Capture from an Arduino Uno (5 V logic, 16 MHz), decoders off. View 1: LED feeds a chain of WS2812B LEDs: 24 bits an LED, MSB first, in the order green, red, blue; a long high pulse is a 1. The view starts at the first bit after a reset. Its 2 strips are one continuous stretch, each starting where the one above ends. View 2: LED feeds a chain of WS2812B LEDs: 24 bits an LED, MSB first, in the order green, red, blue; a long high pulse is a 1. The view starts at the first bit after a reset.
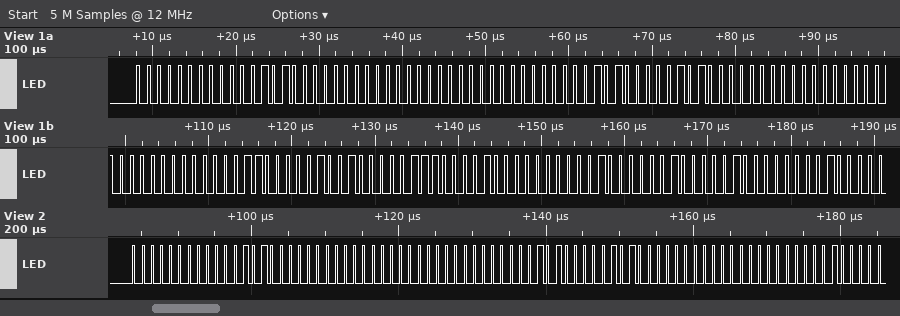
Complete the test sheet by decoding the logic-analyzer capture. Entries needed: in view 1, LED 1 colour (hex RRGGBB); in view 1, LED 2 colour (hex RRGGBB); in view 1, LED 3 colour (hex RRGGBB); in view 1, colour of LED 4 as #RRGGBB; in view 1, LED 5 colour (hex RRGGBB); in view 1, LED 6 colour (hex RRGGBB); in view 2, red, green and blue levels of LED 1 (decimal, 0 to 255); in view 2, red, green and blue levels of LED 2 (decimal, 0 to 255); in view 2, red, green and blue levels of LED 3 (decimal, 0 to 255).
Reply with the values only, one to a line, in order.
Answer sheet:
#0A0000
#00000A
#000A00
#060009
#080701
#080204
10, 0, 0
0, 0, 10
0, 10, 0
